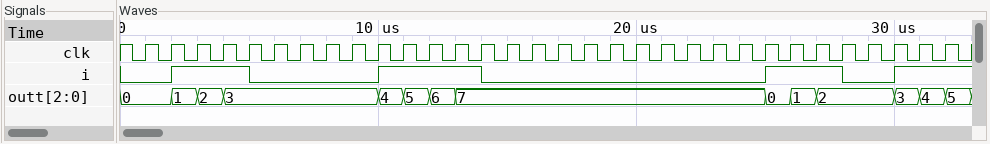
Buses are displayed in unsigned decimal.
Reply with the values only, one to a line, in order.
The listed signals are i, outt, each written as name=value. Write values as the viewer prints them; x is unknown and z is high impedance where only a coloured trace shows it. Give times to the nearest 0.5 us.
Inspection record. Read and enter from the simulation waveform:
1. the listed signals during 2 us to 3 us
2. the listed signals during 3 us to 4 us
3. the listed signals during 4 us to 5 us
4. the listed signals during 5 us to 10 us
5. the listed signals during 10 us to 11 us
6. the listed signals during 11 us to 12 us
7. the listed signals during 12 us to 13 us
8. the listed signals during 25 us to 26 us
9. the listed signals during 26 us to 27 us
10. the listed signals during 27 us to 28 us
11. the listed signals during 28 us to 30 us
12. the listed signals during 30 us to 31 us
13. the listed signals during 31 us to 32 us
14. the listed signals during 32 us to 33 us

i=1, outt=1
i=1, outt=2
i=1, outt=3
i=0, outt=3
i=1, outt=4
i=1, outt=5
i=1, outt=6
i=1, outt=0
i=1, outt=1
i=1, outt=2
i=0, outt=2
i=1, outt=3
i=1, outt=4
i=1, outt=5
